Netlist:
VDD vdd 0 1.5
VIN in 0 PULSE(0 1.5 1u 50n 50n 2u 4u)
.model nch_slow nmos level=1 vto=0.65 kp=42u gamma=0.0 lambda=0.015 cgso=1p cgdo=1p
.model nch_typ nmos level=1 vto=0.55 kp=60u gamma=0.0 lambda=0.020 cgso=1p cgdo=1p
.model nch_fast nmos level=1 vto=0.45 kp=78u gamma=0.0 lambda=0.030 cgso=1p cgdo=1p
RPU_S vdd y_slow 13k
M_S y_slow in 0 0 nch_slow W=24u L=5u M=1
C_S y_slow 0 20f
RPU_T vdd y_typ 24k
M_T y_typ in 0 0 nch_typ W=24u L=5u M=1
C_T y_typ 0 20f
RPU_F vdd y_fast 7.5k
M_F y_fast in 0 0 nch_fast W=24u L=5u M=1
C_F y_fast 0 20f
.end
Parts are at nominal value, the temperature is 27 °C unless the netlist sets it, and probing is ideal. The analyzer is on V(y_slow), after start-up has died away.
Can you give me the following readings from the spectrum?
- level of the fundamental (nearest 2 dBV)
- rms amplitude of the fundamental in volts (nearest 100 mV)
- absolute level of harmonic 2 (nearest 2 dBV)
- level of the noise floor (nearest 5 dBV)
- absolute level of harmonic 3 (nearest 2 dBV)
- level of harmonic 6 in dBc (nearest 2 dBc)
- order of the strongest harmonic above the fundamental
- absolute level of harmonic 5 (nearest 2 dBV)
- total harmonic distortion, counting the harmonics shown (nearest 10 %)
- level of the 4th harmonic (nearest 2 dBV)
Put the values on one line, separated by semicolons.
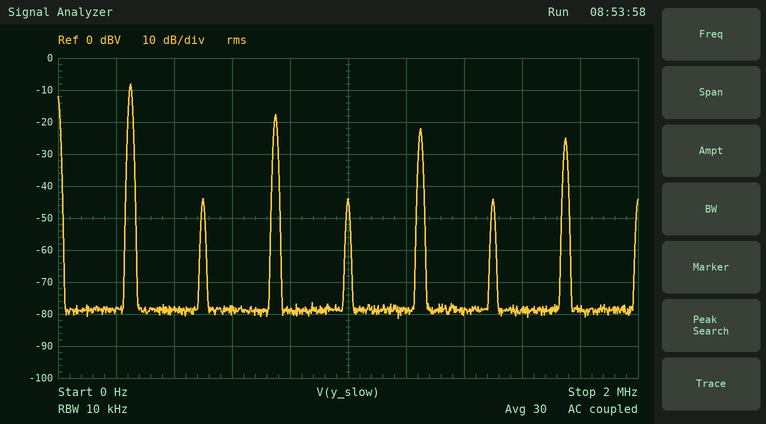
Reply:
-8 dBV; 400 mV; -44 dBV; -80 dBV; -18 dBV; -36 dBc; 3; -22 dBV; 40 %; -44 dBV
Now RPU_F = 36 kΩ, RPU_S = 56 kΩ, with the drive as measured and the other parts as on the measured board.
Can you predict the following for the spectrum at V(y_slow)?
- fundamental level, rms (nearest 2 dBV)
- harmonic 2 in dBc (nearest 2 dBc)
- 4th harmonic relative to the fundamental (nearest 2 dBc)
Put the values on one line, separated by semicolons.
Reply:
-4 dBV; -32 dBc; -32 dBc
